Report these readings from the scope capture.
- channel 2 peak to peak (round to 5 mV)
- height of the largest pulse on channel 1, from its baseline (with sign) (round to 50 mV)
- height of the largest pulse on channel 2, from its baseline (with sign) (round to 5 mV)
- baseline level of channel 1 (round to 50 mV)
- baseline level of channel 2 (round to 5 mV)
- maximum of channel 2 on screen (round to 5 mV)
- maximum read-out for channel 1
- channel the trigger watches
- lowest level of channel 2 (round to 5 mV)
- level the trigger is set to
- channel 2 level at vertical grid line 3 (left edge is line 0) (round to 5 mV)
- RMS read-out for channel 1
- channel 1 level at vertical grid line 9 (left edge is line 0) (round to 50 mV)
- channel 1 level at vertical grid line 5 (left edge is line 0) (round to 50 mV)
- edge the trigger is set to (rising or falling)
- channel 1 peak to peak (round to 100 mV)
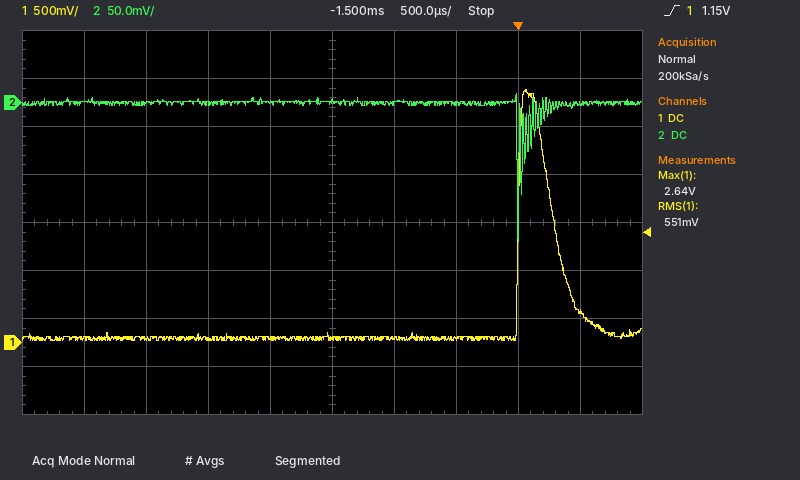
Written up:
155 mV
+2.60 V
-145 mV
50 mV
0 mV
10 mV
2.64 V
channel 1
-145 mV
1.15 V
0 mV
551 mV
300 mV
50 mV
rising
2.60 V
